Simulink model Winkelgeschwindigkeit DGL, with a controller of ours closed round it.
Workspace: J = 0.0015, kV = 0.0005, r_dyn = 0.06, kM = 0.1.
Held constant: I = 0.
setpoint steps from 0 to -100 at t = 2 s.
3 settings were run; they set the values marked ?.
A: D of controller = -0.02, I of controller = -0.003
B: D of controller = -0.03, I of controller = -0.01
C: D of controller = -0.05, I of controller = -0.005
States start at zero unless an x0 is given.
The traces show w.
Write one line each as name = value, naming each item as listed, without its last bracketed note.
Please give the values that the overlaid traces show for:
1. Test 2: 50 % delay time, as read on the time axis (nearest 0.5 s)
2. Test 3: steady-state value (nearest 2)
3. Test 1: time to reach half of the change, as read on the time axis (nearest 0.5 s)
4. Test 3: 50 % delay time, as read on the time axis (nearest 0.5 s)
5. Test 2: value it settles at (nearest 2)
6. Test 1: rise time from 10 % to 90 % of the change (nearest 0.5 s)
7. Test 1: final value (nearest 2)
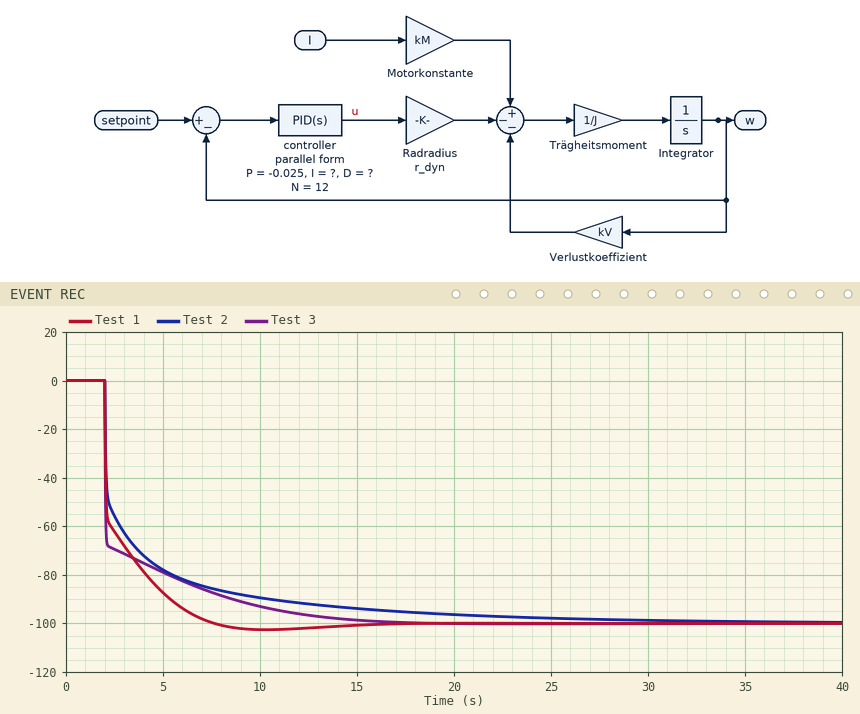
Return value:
Test 2: 50 % delay time, as read on the time axis = 2.0 s
Test 3: steady-state value = -100
Test 1: time to reach half of the change, as read on the time axis = 2.0 s
Test 3: 50 % delay time, as read on the time axis = 2.0 s
Test 2: value it settles at = -100
Test 1: rise time from 10 % to 90 % of the change = 3.5 s
Test 1: final value = -100
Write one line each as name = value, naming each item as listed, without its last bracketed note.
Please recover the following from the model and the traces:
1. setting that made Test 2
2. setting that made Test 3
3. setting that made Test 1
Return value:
setting that made Test 2 = A
setting that made Test 3 = C
setting that made Test 1 = B
